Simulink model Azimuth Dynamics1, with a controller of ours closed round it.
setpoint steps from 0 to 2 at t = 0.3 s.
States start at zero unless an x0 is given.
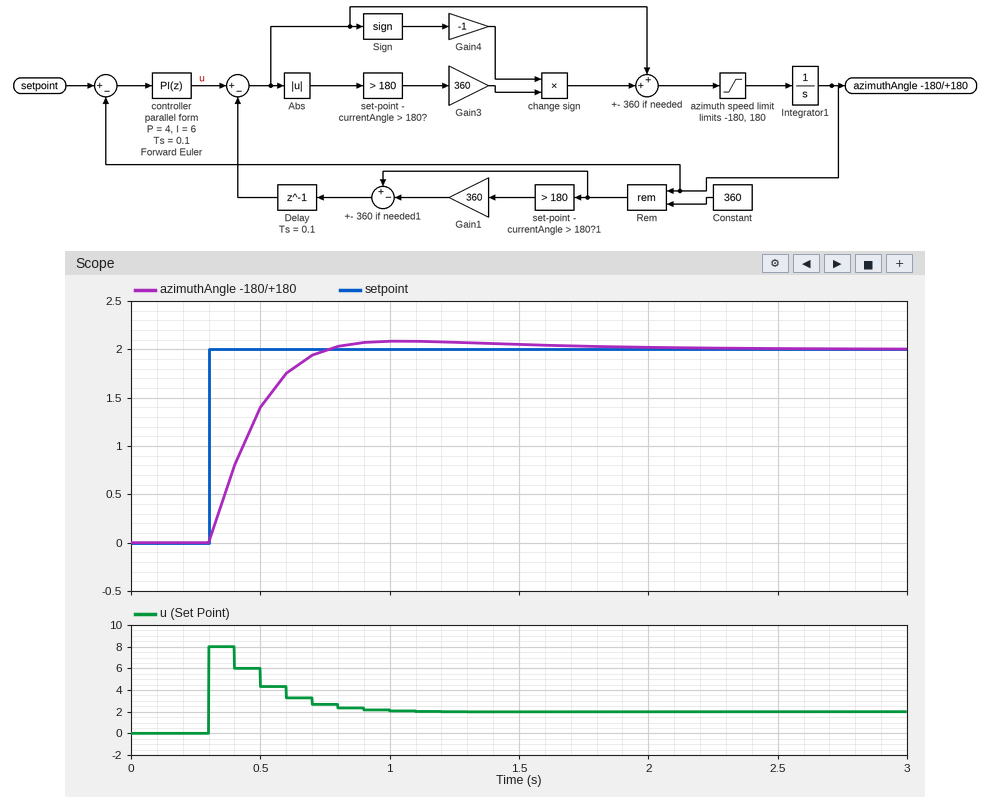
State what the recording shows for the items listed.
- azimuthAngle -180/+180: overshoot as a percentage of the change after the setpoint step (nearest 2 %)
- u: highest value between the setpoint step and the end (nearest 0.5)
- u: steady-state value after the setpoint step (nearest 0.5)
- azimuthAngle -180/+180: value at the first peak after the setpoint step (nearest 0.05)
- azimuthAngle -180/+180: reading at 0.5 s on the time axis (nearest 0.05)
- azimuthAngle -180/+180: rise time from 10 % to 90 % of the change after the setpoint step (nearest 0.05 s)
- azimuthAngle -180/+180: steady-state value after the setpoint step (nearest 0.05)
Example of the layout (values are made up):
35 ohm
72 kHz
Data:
4 %
8.0
2.0
2.10
1.40
0.30 s
2.00
